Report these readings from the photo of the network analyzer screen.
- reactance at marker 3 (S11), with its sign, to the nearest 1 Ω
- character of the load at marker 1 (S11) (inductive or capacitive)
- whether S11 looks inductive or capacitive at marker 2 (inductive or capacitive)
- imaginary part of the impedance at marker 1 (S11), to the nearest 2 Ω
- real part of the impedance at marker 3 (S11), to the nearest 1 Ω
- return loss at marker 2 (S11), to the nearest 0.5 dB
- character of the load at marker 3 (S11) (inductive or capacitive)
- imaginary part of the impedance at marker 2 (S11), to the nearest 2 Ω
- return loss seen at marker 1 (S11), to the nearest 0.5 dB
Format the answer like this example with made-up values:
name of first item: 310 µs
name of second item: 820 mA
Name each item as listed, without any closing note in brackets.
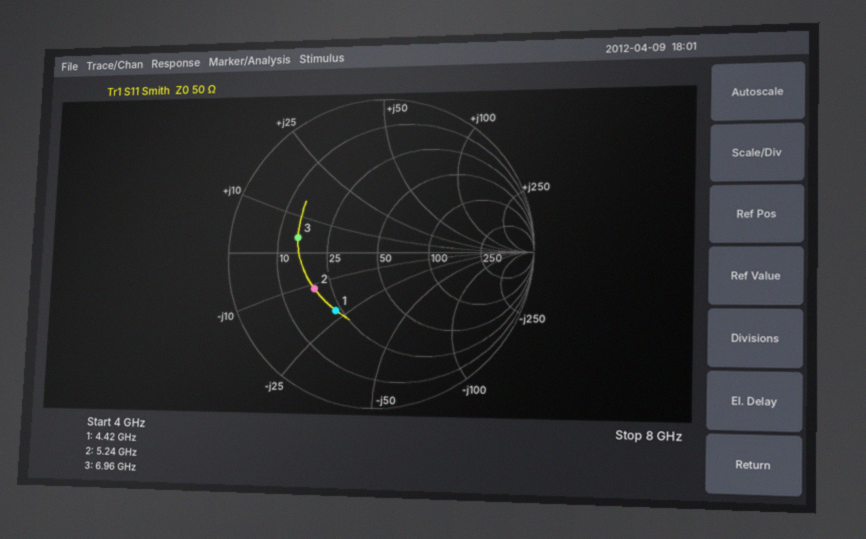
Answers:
reactance at marker 3 (S11), with its sign, to the nearest 1 Ω: +4 Ω
character of the load at marker 1 (S11): capacitive
whether S11 looks inductive or capacitive at marker 2: capacitive
imaginary part of the impedance at marker 1 (S11), to the nearest 2 Ω: -22 Ω
real part of the impedance at marker 3 (S11), to the nearest 1 Ω: 15 Ω
return loss at marker 2 (S11), to the nearest 0.5 dB: 6.5 dB
character of the load at marker 3 (S11): inductive
imaginary part of the impedance at marker 2 (S11), to the nearest 2 Ω: -12 Ω
return loss seen at marker 1 (S11), to the nearest 0.5 dB: 7.0 dB
